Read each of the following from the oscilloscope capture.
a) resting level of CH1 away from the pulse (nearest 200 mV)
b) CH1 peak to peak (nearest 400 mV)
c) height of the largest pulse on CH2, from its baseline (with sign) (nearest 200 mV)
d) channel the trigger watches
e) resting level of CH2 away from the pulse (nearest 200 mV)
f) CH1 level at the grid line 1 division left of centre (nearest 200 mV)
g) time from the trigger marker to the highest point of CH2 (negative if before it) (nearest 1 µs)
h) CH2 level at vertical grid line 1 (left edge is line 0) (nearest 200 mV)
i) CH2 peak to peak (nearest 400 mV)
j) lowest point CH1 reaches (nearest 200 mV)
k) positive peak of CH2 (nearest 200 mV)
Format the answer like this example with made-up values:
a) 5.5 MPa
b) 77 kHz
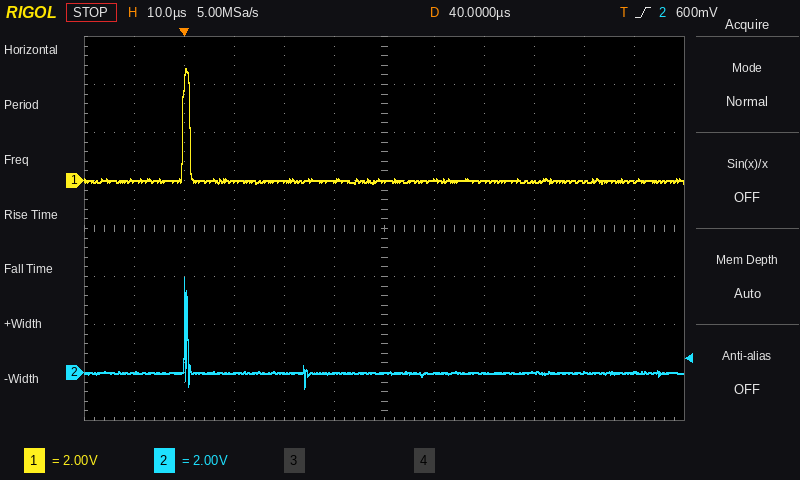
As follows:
a) 0.0 V
b) 4.8 V
c) +4.0 V
d) CH2
e) 0.0 V
f) 0.0 V
g) 0 µs
h) 0.0 V
i) 4.8 V
j) -200 mV
k) 4.0 V
